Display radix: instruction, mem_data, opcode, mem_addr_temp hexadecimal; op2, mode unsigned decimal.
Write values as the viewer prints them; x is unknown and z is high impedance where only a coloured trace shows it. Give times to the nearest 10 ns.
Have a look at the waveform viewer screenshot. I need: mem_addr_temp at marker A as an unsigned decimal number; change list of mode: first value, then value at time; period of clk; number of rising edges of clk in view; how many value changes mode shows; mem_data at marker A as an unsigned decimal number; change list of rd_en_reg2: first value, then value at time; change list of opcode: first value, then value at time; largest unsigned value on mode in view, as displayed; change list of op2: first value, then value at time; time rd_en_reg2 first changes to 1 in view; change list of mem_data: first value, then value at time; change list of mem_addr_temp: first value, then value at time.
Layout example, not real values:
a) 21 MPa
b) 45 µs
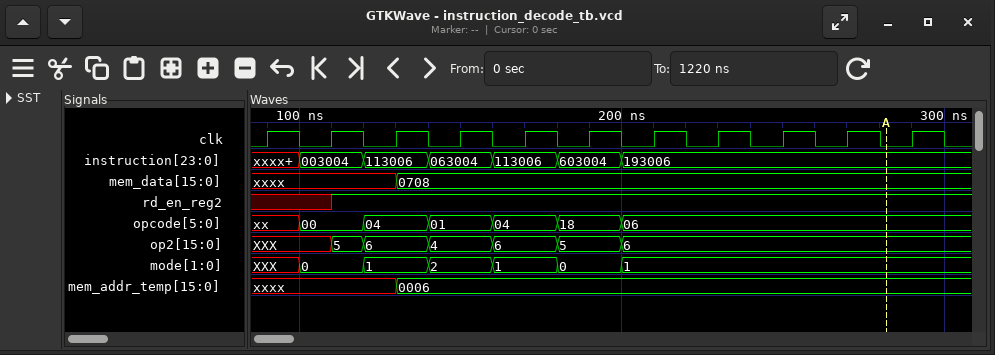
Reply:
a) 6
b) XXX, 0 at 100 ns, 1 at 120 ns, 2 at 140 ns, 1 at 160 ns, 0 at 180 ns, 1 at 200 ns
c) 20 ns
d) 11
e) 6
f) 1800
g) x, 1 at 110 ns
h) xx, 00 at 100 ns, 04 at 120 ns, 01 at 140 ns, 04 at 160 ns, 18 at 180 ns, 06 at 200 ns
i) 2
j) XXX, 5 at 110 ns, 6 at 120 ns, 4 at 140 ns, 6 at 160 ns, 5 at 180 ns, 6 at 200 ns
k) 110 ns
l) xxxx, 0708 at 130 ns
m) xxxx, 0006 at 130 ns
